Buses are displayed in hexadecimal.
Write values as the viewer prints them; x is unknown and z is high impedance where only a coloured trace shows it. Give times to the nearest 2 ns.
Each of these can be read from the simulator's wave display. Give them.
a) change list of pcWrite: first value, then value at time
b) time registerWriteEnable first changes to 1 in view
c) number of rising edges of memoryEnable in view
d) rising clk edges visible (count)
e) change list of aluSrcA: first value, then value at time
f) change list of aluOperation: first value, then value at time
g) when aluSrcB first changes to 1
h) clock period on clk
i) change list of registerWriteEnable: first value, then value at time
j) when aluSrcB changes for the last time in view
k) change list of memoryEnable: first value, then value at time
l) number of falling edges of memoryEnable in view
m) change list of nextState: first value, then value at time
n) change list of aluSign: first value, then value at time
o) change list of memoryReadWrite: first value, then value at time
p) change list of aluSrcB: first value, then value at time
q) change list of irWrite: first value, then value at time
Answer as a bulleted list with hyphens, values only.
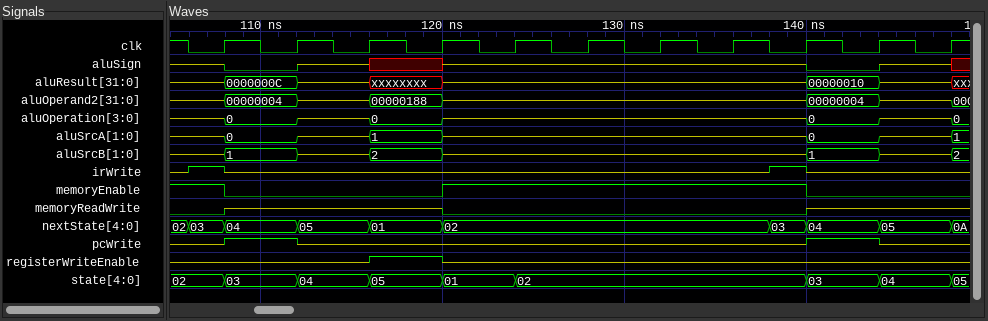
- z, 1 at 108 ns, z at 112 ns, 1 at 140 ns, z at 144 ns
- 116 ns
- 1
- 11
- z, 0 at 108 ns, z at 112 ns, 1 at 116 ns, z at 120 ns, 0 at 140 ns, z at 144 ns, 1 at 148 ns
- z, 0 at 108 ns, z at 112 ns, 0 at 116 ns, z at 120 ns, 0 at 140 ns, z at 144 ns, 0 at 148 ns
- 108 ns
- 4 ns
- z, 1 at 116 ns, z at 120 ns
- 148 ns
- 1, 0 at 108 ns, 1 at 120 ns, 0 at 140 ns
- 2
- 02, 03 at 106 ns, 04 at 108 ns, 05 at 112 ns, 01 at 116 ns, 02 at 120 ns, 03 at 138 ns, 04 at 140 ns, 05 at 144 ns, 0A at 148 ns
- z, 0 at 108 ns, z at 112 ns, x at 116 ns, z at 120 ns, 0 at 140 ns, z at 144 ns, x at 148 ns
- 0, z at 108 ns, 0 at 120 ns, z at 140 ns
- z, 1 at 108 ns, z at 112 ns, 2 at 116 ns, z at 120 ns, 1 at 140 ns, z at 144 ns, 2 at 148 ns
- z, 1 at 106 ns, z at 108 ns, 1 at 138 ns, z at 140 ns
